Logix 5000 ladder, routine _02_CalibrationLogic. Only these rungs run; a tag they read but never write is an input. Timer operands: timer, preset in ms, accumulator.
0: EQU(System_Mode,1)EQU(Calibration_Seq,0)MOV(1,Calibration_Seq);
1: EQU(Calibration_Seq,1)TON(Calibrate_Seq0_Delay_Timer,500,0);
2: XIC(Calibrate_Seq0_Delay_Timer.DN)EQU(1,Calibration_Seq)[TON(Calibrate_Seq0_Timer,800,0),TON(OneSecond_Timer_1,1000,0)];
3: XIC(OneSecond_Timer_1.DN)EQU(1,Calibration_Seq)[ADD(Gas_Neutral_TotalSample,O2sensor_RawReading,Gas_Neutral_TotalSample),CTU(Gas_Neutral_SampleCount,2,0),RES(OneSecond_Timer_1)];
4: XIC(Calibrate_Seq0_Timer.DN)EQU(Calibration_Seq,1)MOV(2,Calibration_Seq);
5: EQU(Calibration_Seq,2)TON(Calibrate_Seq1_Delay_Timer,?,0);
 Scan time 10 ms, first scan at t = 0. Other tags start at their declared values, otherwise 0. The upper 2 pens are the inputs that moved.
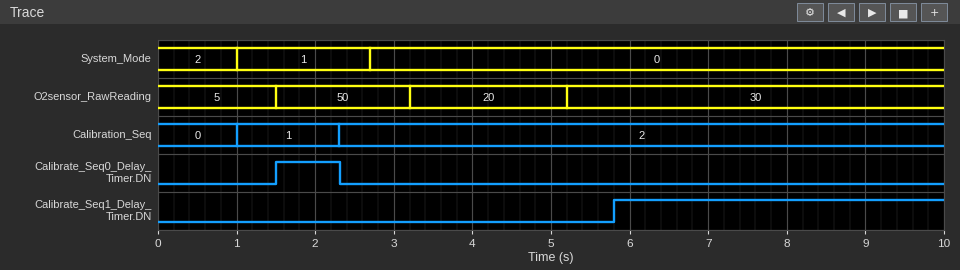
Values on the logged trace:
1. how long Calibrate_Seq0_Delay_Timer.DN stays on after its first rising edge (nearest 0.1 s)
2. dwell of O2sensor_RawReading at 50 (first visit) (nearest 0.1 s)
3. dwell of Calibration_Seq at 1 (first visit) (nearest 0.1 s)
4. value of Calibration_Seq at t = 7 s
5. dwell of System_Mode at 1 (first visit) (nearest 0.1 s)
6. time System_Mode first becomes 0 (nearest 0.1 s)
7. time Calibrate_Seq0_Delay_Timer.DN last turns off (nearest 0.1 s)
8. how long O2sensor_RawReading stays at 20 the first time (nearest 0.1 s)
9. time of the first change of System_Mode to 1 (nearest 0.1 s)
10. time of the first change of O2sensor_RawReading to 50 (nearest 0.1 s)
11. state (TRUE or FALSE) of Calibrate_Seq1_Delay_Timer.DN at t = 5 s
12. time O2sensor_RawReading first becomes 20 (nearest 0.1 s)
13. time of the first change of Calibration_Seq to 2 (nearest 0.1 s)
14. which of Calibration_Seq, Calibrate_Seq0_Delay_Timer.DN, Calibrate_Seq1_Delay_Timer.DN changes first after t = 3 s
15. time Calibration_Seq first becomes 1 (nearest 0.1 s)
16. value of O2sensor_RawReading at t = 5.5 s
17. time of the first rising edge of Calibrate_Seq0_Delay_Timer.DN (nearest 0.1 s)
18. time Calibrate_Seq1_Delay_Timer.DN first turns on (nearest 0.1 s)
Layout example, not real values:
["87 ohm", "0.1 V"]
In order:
["0.8 s", "1.7 s", "1.3 s", "2", "1.7 s", "2.7 s", "2.3 s", "2.0 s", "1.0 s", "1.5 s", "FALSE", "3.2 s", "2.3 s", "Calibrate_Seq1_Delay_Timer.DN", "1.0 s", "30", "1.5 s", "5.8 s"]
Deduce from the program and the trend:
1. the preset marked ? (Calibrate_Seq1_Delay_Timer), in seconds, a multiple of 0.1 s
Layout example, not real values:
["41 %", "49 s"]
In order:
["3.5 s"]
